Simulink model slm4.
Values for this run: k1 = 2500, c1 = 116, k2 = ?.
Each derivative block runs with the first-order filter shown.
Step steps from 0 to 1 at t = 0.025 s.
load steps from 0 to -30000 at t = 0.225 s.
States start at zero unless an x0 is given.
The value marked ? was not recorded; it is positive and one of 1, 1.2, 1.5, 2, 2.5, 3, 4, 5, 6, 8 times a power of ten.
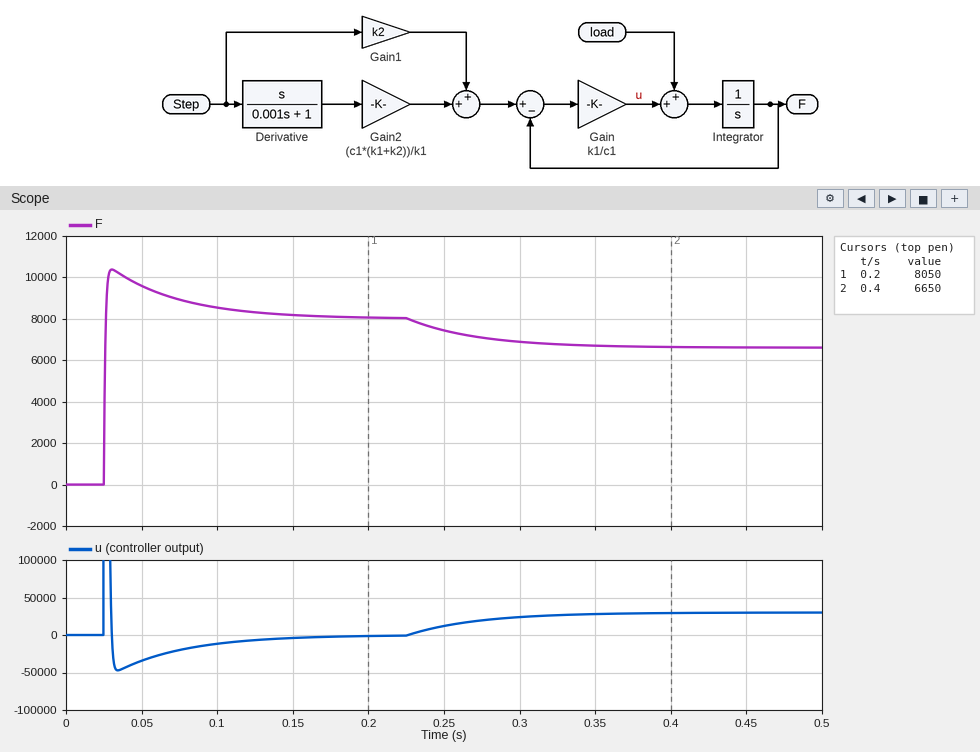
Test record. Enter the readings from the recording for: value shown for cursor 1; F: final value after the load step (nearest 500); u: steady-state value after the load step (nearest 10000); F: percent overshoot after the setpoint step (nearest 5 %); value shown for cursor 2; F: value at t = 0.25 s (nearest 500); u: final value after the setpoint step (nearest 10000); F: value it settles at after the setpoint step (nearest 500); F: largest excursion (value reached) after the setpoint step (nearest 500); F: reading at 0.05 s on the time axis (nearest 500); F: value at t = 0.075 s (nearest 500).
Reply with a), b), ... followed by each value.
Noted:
a) 8050
b) 6500
c) 30000
d) 30 %
e) 6650
f) 7500
g) 0
h) 8000
i) 10500
j) 9500
k) 9000
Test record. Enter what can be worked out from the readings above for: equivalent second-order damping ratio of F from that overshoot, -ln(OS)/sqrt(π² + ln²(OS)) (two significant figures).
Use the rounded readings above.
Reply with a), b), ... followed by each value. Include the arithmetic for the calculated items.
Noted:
a) ln(0.3) = -1.204; 1.204 / sqrt(9.870 + 1.450) = 0.36
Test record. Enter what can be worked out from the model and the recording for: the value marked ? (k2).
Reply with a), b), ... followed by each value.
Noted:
a) 8000
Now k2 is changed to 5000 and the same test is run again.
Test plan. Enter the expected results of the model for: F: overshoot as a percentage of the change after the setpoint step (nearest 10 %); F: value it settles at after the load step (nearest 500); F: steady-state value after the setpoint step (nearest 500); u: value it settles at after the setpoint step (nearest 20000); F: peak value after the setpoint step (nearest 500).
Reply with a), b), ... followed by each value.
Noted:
a) 50 %
b) 3500
c) 5000
d) 0
e) 7500
